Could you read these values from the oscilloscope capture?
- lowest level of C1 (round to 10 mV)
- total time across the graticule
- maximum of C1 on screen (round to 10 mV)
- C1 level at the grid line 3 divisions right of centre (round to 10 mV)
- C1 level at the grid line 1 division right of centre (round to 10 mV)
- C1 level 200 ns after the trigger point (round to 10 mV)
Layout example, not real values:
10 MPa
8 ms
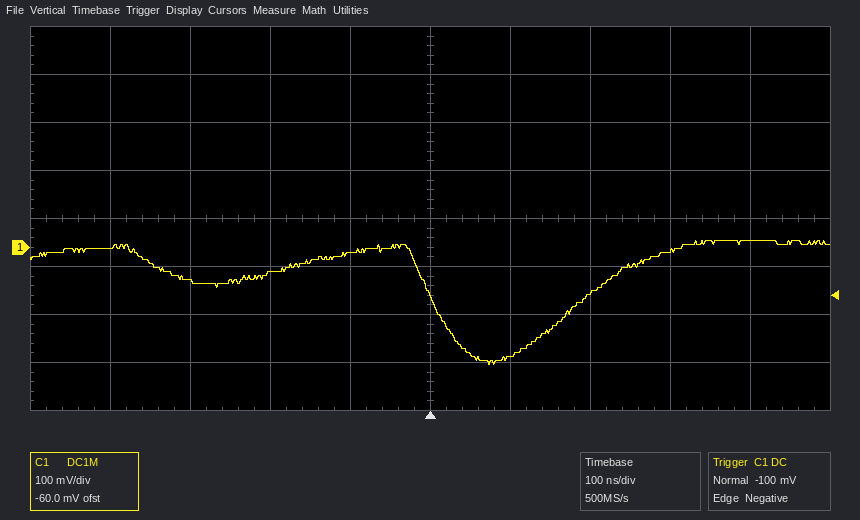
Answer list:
-240 mV
1 µs
10 mV
-10 mV
-230 mV
-100 mV
